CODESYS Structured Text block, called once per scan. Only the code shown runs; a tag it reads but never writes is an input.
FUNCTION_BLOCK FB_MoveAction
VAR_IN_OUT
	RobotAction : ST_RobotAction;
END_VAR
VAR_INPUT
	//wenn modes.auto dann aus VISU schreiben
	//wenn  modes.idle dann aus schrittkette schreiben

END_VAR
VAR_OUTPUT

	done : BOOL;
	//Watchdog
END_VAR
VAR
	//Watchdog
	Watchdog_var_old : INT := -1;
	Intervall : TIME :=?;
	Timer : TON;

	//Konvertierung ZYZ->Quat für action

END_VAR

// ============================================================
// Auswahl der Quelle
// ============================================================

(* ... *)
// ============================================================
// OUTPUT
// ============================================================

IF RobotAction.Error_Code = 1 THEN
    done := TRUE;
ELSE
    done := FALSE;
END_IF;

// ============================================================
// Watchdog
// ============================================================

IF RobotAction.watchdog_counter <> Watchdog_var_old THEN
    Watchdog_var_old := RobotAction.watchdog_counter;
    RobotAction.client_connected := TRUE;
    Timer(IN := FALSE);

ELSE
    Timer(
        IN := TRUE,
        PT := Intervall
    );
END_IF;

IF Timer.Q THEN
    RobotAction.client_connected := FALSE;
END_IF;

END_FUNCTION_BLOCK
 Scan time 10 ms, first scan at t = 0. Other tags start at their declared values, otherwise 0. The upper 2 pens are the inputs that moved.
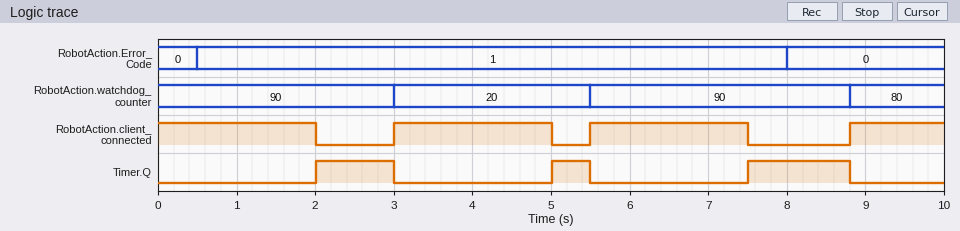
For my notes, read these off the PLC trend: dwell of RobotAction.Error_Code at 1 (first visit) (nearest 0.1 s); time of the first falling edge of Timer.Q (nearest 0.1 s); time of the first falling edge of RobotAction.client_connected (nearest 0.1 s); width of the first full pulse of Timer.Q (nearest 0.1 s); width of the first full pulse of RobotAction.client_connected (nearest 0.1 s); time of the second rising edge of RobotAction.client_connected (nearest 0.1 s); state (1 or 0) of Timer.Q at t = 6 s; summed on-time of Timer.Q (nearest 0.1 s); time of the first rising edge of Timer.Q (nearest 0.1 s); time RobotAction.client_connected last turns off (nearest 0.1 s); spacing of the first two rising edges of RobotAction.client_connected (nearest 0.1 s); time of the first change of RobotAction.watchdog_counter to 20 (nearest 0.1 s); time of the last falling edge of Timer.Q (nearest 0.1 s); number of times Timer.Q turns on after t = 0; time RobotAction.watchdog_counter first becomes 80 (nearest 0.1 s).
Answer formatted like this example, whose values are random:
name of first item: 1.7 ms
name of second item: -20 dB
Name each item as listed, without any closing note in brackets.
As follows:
dwell of RobotAction.Error_Code at 1 (first visit): 7.5 s
time of the first falling edge of Timer.Q: 3.0 s
time of the first falling edge of RobotAction.client_connected: 2.0 s
width of the first full pulse of Timer.Q: 1.0 s
width of the first full pulse of RobotAction.client_connected: 2.0 s
time of the second rising edge of RobotAction.client_connected: 5.5 s
state (1 or 0) of Timer.Q at t = 6 s: 0
summed on-time of Timer.Q: 2.8 s
time of the first rising edge of Timer.Q: 2.0 s
time RobotAction.client_connected last turns off: 7.5 s
spacing of the first two rising edges of RobotAction.client_connected: 2.5 s
time of the first change of RobotAction.watchdog_counter to 20: 3.0 s
time of the last falling edge of Timer.Q: 8.8 s
number of times Timer.Q turns on after t = 0: 3
time RobotAction.watchdog_counter first becomes 80: 8.8 s
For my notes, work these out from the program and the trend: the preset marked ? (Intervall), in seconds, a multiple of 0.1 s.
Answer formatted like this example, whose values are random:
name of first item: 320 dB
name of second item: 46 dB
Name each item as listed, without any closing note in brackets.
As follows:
the preset marked ? (Intervall), in seconds, a multiple of 0.1 s: 2.0 s
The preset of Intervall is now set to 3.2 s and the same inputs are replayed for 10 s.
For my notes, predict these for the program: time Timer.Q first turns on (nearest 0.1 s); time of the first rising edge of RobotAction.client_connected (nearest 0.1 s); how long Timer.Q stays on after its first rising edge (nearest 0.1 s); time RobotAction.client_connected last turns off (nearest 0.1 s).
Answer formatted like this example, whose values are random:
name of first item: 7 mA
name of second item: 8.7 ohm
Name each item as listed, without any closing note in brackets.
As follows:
time Timer.Q first turns on: 8.7 s
time of the first rising edge of RobotAction.client_connected: 8.8 s
how long Timer.Q stays on after its first rising edge: 0.1 s
time RobotAction.client_connected last turns off: 8.7 s
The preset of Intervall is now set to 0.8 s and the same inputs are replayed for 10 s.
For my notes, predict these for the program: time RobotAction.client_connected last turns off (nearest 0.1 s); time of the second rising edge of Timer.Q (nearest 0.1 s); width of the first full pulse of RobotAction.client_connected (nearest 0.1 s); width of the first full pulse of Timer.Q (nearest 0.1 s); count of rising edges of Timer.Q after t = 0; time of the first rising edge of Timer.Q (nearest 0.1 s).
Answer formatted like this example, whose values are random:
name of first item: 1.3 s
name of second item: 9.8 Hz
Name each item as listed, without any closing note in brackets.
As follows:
time RobotAction.client_connected last turns off: 9.6 s
time of the second rising edge of Timer.Q: 3.8 s
width of the first full pulse of RobotAction.client_connected: 0.8 s
width of the first full pulse of Timer.Q: 2.2 s
count of rising edges of Timer.Q after t = 0: 4
time of the first rising edge of Timer.Q: 0.8 s
